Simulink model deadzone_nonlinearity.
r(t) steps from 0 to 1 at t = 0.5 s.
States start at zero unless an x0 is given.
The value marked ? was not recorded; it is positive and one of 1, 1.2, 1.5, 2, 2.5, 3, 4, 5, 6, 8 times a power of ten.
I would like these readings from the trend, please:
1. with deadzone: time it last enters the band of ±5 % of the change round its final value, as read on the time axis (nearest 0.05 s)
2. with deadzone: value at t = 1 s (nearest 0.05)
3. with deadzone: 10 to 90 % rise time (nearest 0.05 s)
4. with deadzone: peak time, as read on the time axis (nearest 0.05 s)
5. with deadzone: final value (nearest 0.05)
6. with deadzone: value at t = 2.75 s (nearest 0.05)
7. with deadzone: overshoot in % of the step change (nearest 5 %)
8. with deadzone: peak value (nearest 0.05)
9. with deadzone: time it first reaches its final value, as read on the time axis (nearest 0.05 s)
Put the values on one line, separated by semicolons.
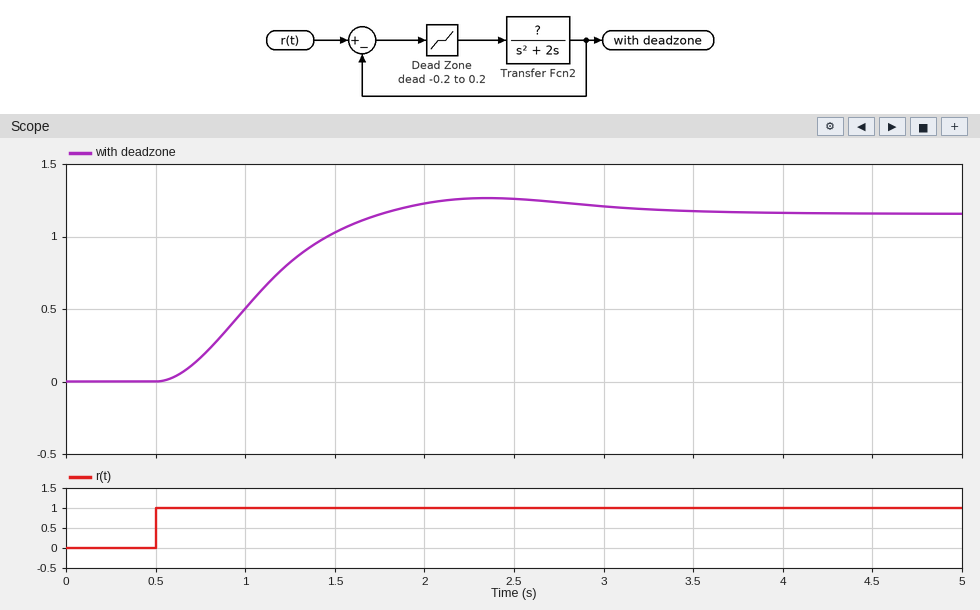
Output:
2.95 s; 0.50; 0.80 s; 2.35 s; 1.15; 1.25; 10 %; 1.25; 1.75 s
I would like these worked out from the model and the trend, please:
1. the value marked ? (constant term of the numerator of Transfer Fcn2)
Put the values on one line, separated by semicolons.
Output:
8
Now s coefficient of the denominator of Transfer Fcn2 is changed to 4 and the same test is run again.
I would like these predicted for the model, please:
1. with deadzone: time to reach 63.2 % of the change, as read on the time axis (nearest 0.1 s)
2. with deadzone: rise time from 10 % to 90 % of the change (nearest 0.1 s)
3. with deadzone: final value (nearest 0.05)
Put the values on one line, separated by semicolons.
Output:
1.2 s; 0.9 s; 0.85
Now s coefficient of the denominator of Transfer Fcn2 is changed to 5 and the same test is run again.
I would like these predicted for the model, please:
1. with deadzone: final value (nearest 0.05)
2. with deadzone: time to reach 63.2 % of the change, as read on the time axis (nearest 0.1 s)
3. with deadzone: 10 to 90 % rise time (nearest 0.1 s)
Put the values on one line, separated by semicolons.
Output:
0.80; 1.2 s; 1.0 s
